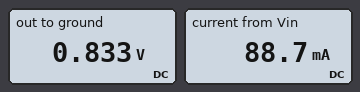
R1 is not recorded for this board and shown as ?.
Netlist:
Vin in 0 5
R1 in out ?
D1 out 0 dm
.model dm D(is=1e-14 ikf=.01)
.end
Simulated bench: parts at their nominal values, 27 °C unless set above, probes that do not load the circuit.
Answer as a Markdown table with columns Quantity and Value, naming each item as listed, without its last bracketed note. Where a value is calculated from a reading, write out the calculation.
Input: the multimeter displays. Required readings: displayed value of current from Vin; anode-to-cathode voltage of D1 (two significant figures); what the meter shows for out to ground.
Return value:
| Quantity | Value |
|---|---|
| displayed value of current from Vin | 88.7 mA |
| anode-to-cathode voltage of D1 | 833 mV = 830 mV |
| what the meter shows for out to ground | 0.833 V |
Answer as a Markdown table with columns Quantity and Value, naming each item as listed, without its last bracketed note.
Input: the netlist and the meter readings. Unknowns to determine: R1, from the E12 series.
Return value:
| Quantity | Value |
|---|---|
| R1, from the E12 series | 47 Ω |
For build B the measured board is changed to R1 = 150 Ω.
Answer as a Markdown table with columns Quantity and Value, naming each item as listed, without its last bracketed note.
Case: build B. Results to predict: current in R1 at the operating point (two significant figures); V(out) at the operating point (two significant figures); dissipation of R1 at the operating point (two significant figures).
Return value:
| Quantity | Value |
|---|---|
| current in R1 at the operating point | 28 mA |
| V(out) at the operating point | 780 mV |
| dissipation of R1 at the operating point | 120 mW |
